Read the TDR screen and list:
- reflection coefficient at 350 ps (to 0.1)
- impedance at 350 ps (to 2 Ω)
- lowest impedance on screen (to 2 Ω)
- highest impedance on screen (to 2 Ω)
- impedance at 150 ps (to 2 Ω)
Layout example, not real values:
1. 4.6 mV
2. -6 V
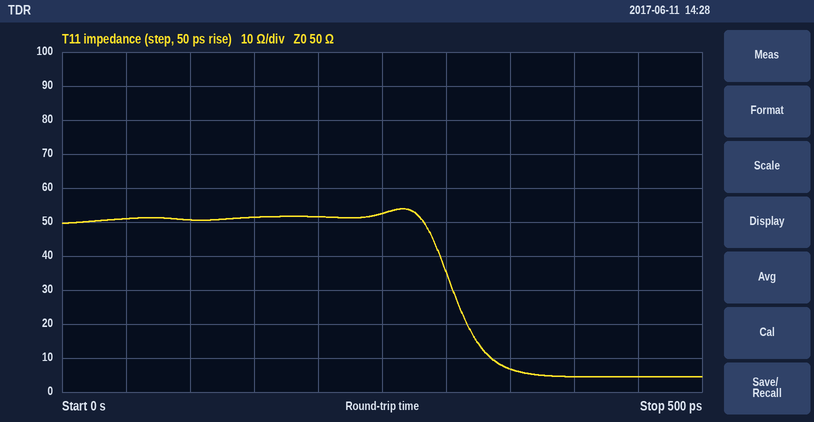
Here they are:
1. -0.8
2. 6 Ω
3. 4 Ω
4. 54 Ω
5. 52 Ω
